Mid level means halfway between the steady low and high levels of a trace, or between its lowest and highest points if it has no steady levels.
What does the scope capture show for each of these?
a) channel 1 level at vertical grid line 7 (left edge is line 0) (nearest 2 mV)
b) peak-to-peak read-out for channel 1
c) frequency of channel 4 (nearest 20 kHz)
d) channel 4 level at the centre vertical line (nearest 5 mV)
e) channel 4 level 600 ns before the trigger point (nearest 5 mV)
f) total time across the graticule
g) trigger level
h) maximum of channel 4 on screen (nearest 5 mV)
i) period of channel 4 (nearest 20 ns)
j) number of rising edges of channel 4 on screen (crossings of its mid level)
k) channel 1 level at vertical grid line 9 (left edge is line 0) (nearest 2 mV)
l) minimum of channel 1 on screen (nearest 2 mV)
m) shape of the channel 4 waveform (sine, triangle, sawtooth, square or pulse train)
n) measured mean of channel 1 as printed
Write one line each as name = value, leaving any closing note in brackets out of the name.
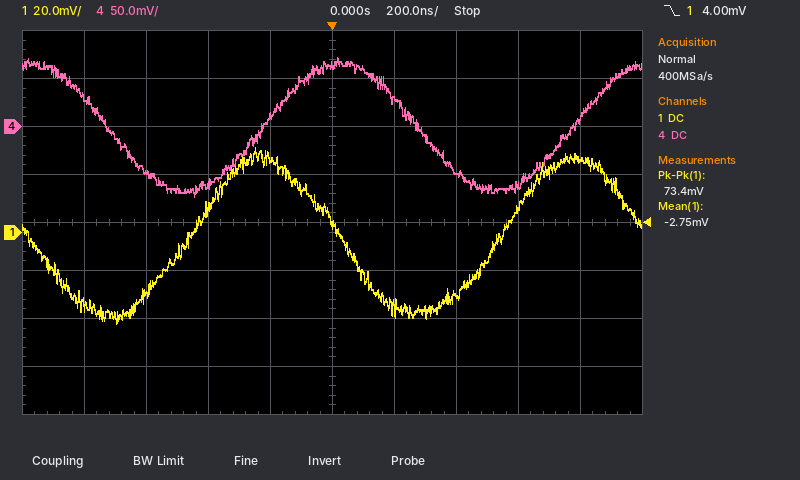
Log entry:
channel 1 level at vertical grid line 7 (left edge is line 0) = -26 mV
peak-to-peak read-out for channel 1 = 73.4 mV
frequency of channel 4 = 1.00 MHz
channel 4 level at the centre vertical line = 65 mV
channel 4 level 600 ns before the trigger point = -50 mV
total time across the graticule = 2 µs
trigger level = 4.00 mV
maximum of channel 4 on screen = 70 mV
period of channel 4 = 1.00 µs
number of rising edges of channel 4 on screen = 2
channel 1 level at vertical grid line 9 (left edge is line 0) = 30 mV
minimum of channel 1 on screen = -38 mV
shape of the channel 4 waveform = sine
measured mean of channel 1 as printed = -2.75 mV
